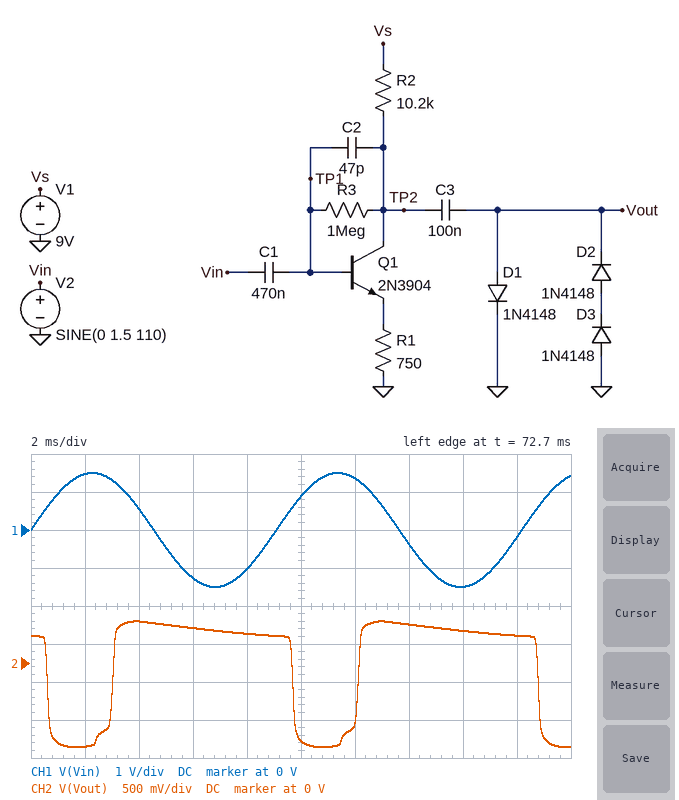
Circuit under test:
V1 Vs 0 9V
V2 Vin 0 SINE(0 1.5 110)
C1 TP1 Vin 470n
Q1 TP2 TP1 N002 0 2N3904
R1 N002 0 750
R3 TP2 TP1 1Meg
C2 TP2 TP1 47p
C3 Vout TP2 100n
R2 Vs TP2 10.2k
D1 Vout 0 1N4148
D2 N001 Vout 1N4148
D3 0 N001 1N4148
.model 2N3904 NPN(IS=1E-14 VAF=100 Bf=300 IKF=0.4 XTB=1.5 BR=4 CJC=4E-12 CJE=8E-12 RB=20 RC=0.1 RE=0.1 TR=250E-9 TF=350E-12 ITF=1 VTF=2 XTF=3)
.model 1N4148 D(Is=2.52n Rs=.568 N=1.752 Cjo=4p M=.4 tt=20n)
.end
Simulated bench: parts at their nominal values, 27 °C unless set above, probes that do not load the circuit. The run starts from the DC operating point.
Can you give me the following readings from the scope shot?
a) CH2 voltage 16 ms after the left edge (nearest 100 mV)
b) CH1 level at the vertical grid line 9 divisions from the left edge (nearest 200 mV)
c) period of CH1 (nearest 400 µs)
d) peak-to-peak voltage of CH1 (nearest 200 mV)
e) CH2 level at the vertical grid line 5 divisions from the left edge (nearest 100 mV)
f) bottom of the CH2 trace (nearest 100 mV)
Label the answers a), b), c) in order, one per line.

a) 400 mV
b) -200 mV
c) 9.2 ms
d) 3.0 V
e) -1.0 V
f) -1.1 V
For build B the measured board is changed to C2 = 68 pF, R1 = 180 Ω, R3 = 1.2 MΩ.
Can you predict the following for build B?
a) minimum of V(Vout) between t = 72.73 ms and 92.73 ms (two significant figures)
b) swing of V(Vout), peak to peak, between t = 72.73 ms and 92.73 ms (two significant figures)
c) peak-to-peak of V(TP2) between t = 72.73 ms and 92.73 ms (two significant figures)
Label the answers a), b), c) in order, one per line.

a) -1.2 V
b) 1.7 V
c) 8.7 V
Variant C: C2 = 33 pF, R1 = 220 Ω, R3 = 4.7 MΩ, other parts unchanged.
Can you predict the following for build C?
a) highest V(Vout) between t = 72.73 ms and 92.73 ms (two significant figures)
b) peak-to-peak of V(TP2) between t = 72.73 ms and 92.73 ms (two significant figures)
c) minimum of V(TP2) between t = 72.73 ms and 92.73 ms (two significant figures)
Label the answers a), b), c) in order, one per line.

a) 560 mV
b) 8.7 V
c) 260 mV
